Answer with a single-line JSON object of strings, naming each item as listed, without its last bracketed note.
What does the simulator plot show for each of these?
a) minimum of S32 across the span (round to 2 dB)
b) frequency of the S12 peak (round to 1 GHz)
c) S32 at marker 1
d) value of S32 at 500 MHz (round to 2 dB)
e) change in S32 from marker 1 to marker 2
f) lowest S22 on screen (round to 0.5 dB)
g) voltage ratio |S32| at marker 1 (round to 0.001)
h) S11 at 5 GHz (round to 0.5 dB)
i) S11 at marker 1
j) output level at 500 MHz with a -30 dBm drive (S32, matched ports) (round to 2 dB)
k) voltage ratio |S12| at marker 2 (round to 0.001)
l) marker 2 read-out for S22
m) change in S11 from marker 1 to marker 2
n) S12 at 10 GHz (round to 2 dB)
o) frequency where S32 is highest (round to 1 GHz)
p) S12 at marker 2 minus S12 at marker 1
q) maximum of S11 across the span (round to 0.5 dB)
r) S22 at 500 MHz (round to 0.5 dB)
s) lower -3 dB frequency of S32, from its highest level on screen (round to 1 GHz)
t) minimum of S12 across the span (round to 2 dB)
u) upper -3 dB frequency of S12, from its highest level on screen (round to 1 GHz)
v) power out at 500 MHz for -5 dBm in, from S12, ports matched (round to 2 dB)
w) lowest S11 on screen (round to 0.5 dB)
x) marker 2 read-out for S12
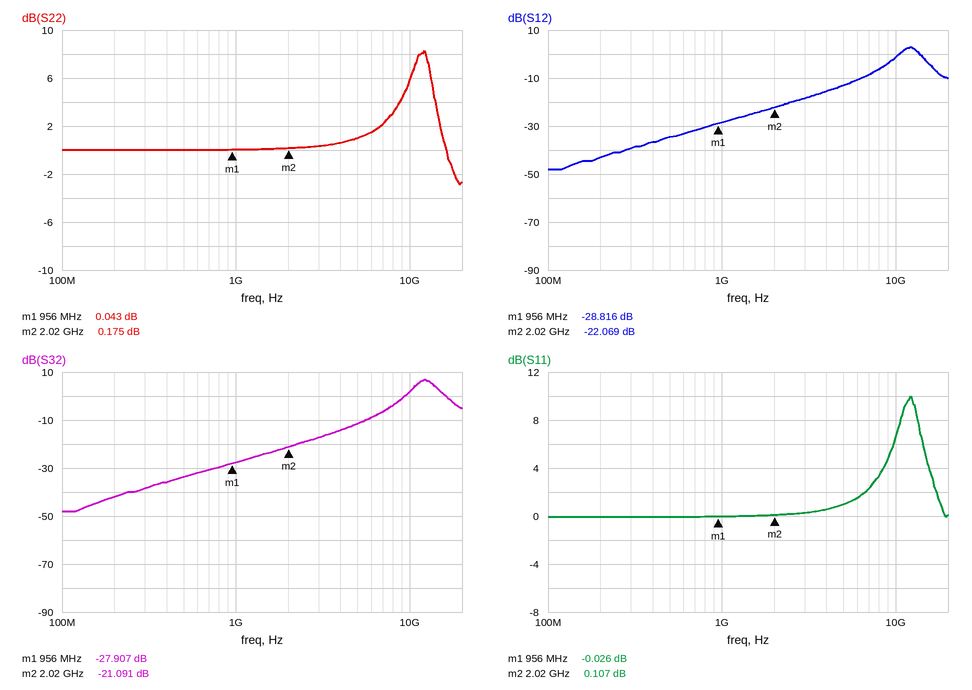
{"minimum of S32 across the span": "-48 dB", "frequency of the S12 peak": "12 GHz", "S32 at marker 1": "-27.907 dB", "value of S32 at 500 MHz": "-34 dB", "change in S32 from marker 1 to marker 2": "6.816 dB", "lowest S22 on screen": "-3.0 dB", "voltage ratio |S32| at marker 1": "0.040", "S11 at 5 GHz": "1.0 dB", "S11 at marker 1": "-0.026 dB", "output level at 500 MHz with a -30 dBm drive (S32, matched ports)": "-64 dBm", "voltage ratio |S12| at marker 2": "0.079", "marker 2 read-out for S22": "0.175 dB", "change in S11 from marker 1 to marker 2": "0.133 dB", "S12 at 10 GHz": "-2 dB", "frequency where S32 is highest": "12 GHz", "S12 at marker 2 minus S12 at marker 1": "6.747 dB", "maximum of S11 across the span": "10.0 dB", "S22 at 500 MHz": "0.0 dB", "lower -3 dB frequency of S32, from its highest level on screen": "11 GHz", "minimum of S12 across the span": "-48 dB", "upper -3 dB frequency of S12, from its highest level on screen": "14 GHz", "power out at 500 MHz for -5 dBm in, from S12, ports matched": "-40 dBm", "lowest S11 on screen": "0.0 dB", "marker 2 read-out for S12": "-22.069 dB"}
